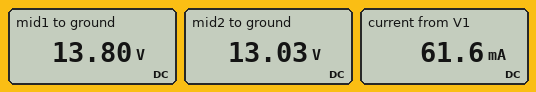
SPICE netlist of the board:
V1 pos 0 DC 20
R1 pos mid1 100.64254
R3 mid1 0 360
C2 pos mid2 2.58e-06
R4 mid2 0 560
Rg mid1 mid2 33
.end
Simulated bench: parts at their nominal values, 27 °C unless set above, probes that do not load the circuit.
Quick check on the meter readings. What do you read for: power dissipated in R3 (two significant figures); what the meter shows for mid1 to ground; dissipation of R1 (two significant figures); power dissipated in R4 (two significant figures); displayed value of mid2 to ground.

530 mW
13.80 V
380 mW
300 mW
13.03 V
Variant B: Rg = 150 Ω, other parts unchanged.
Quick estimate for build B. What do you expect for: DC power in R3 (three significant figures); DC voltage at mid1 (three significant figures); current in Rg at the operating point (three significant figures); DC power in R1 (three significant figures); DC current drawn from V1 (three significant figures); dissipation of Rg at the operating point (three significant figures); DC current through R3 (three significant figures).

550 mW
14.1 V
19.8 mA
349 mW
58.9 mA
58.9 mW
39.1 mA
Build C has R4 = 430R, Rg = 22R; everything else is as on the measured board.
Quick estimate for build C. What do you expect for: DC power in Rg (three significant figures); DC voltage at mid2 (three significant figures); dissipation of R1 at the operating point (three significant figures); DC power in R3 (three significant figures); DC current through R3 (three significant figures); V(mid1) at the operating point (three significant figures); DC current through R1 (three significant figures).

19.1 mW
12.7 V
444 mW
492 mW
37.0 mA
13.3 V
66.4 mA
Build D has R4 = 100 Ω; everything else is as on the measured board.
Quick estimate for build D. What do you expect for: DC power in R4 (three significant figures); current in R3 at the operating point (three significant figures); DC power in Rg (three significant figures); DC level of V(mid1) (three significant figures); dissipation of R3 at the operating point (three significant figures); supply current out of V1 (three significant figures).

545 mW
27.3 mA
180 mW
9.82 V
268 mW
101 mA
